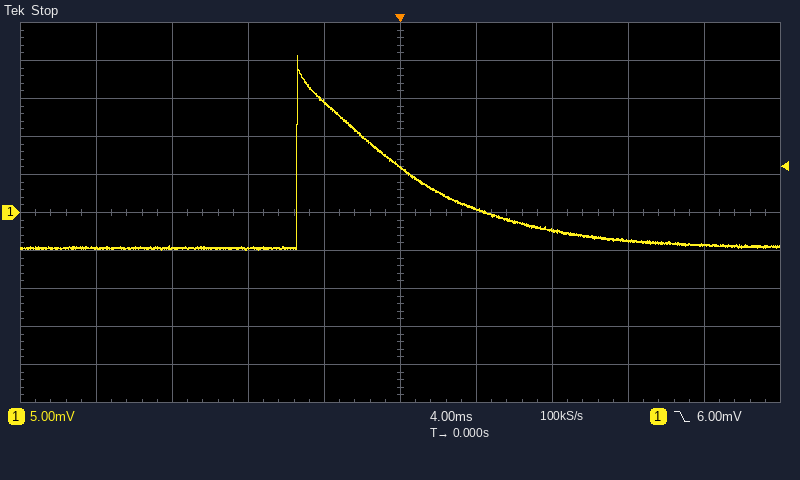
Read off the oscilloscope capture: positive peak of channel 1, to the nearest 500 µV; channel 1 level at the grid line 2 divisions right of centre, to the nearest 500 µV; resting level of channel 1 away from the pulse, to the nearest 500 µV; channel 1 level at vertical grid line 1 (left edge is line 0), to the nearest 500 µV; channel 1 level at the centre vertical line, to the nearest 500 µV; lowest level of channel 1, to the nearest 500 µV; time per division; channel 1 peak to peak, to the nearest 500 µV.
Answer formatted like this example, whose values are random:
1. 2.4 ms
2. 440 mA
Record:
1. 20.5 mV
2. -2.5 mV
3. -4.5 mV
4. -4.5 mV
5. 6.0 mV
6. -5.0 mV
7. 4 ms
8. 25.5 mV
